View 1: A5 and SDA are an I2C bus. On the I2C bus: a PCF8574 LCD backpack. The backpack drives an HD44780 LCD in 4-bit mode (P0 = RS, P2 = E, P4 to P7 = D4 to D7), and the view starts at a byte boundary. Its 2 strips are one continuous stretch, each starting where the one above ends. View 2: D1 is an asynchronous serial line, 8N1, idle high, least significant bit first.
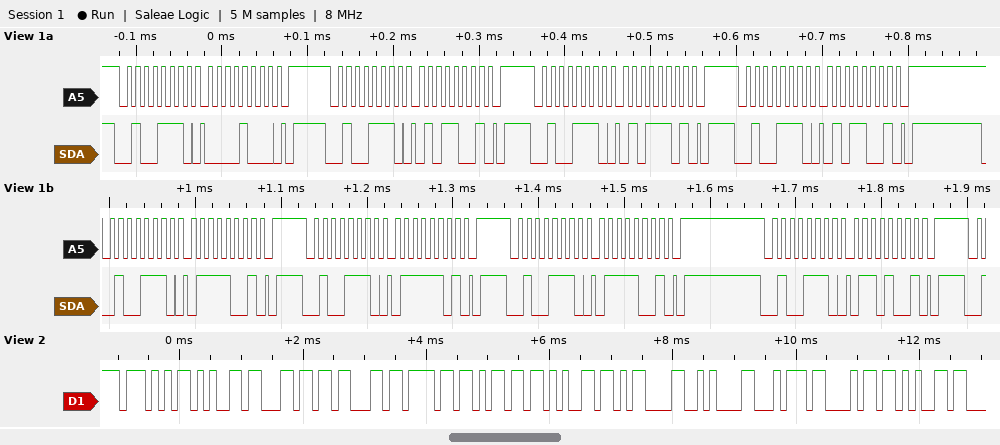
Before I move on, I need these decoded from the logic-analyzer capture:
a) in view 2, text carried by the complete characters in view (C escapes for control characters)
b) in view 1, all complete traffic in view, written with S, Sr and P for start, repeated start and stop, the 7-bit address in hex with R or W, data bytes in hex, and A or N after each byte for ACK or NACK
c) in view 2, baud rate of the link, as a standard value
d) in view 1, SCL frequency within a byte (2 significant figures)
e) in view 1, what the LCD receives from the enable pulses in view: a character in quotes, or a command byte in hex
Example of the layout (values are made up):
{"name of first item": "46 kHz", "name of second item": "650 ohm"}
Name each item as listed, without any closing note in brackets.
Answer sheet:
{"in view 2, text carried by the complete characters in view": "\"Welcome\\r\\nthe\"", "in view 1, all complete traffic in view, written with S, Sr and P for start, repeated start and stop, the 7-bit address in hex with R or W, data bytes in hex, and A or N after each byte for ACK or NACK": "S 27W A 08 A P S 27W A 59 A P S 27W A 5D A P S 27W A 59 A P S 27W A 79 A P S 27W A 7D A P S 27W A 79 A P S 27W A 69 A P", "in view 2, baud rate of the link, as a standard value": "9600 baud", "in view 1, SCL frequency within a byte": "100 kHz", "in view 1, what the LCD receives from the enable pulses in view: a character in quotes, or a command byte in hex": "'W'"}
